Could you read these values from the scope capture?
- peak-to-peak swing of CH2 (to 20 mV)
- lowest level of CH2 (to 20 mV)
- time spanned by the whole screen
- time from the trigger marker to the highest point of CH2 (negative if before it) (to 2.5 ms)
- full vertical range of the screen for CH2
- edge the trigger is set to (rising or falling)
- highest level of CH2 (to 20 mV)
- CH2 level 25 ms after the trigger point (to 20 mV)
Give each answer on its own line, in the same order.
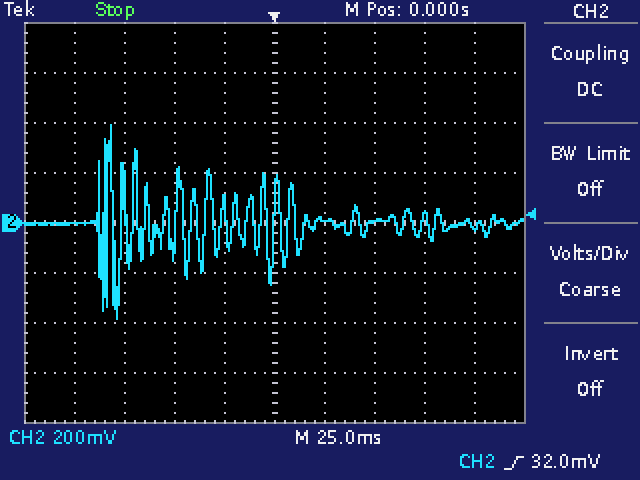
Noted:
780 mV
-380 mV
250 ms
-82.5 ms
1.6 V
rising
400 mV
20 mV
